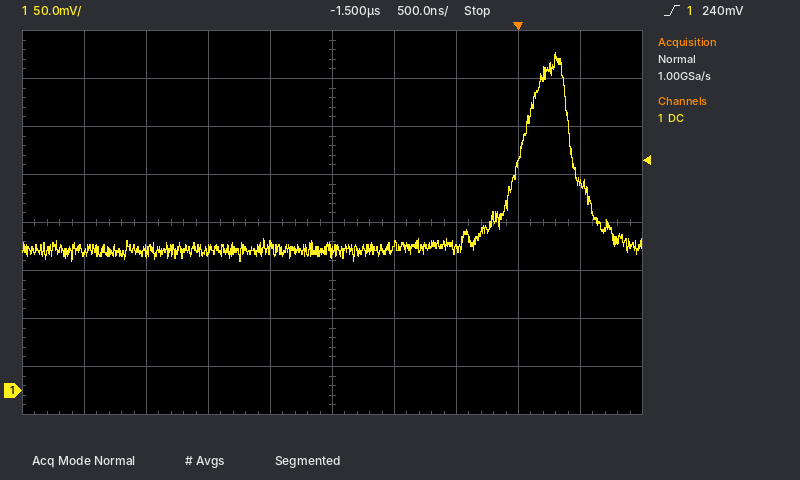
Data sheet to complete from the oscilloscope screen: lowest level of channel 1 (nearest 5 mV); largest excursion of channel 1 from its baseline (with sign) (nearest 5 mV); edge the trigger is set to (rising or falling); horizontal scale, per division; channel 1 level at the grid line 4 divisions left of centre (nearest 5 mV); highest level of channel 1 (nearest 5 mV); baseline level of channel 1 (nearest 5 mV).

135 mV
+205 mV
rising
500 ns
145 mV
350 mV
145 mV
